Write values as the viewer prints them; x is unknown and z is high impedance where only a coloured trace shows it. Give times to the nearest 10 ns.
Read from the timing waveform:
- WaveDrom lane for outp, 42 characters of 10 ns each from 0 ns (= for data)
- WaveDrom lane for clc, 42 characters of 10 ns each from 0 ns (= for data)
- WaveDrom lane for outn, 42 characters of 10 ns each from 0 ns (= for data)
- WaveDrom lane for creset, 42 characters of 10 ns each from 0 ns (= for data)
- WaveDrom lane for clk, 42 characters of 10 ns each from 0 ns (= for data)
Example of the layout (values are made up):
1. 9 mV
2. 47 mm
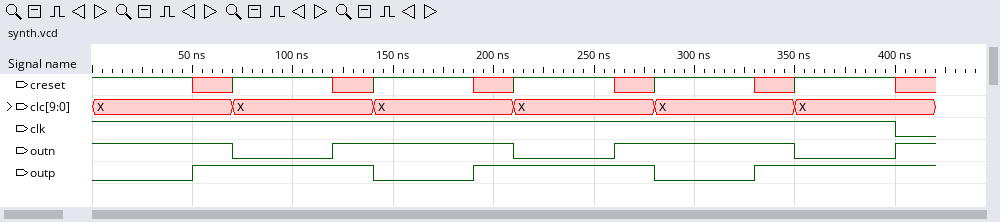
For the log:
1. {name: 'outp', wave: '0....1........0....1........0....1........'}
2. {name: 'clc', wave: '=......=......=......=......=......=......', data: 'X X X X X X'}
3. {name: 'outn', wave: '1......0....1........0....1........0....1.'}
4. {name: 'creset', wave: '1....x.1....x.1....x.1....x.1....x.1....x.'}
5. {name: 'clk', wave: '1.......................................0.'}
